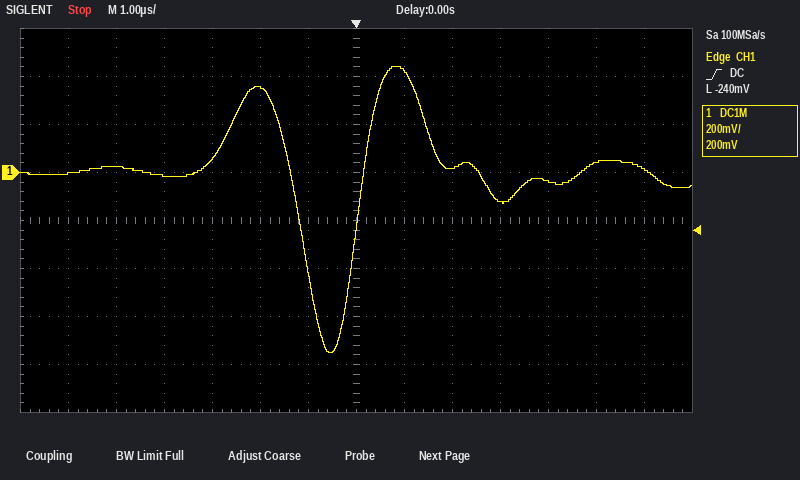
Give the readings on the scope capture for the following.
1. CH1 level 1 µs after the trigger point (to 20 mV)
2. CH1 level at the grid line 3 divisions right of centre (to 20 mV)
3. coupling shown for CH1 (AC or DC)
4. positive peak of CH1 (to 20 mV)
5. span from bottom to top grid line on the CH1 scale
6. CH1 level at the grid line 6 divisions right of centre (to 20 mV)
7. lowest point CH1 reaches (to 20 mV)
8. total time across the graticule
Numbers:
420 mV
-120 mV
DC
440 mV
1.6 V
20 mV
-760 mV
14 µs
